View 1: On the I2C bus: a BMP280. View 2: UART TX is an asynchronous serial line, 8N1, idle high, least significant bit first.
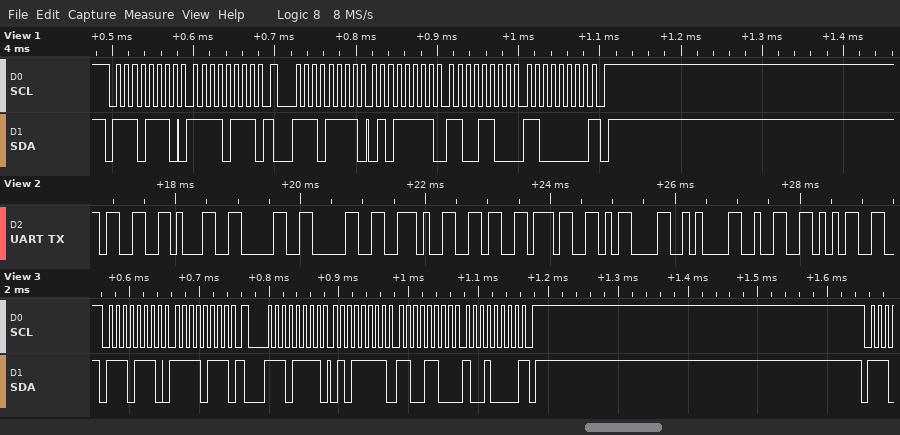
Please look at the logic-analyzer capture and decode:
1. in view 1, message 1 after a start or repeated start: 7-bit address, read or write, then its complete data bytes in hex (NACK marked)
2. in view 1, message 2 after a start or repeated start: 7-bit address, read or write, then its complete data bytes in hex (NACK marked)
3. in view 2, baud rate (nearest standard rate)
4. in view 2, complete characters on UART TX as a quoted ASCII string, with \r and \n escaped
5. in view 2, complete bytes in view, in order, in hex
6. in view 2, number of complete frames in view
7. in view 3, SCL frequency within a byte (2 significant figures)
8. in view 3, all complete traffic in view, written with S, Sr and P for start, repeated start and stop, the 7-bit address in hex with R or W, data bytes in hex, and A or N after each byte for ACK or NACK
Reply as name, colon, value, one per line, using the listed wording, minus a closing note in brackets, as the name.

in view 1, message 1 after a start or repeated start: 7-bit address, read or write, then its complete data bytes in hex: 0x77 write: F7
in view 1, message 2 after a start or repeated start: 7-bit address, read or write, then its complete data bytes in hex: 0x77 read: 5F CC C0 NACK
in view 2, baud rate: 9600 baud
in view 2, complete characters on UART TX as a quoted ASCII string, with \r and \n escaped: "3100.67\r\n25"
in view 2, complete bytes in view, in order, in hex: 33 31 30 30 2E 36 37 0D 0A 32 35
in view 2, number of complete frames in view: 11
in view 3, SCL frequency within a byte: 100 kHz
in view 3, all complete traffic in view, written with S, Sr and P for start, repeated start and stop, the 7-bit address in hex with R or W, data bytes in hex, and A or N after each byte for ACK or NACK: S 77W A F7 A Sr 77R A 5F A CC A 90 N P
